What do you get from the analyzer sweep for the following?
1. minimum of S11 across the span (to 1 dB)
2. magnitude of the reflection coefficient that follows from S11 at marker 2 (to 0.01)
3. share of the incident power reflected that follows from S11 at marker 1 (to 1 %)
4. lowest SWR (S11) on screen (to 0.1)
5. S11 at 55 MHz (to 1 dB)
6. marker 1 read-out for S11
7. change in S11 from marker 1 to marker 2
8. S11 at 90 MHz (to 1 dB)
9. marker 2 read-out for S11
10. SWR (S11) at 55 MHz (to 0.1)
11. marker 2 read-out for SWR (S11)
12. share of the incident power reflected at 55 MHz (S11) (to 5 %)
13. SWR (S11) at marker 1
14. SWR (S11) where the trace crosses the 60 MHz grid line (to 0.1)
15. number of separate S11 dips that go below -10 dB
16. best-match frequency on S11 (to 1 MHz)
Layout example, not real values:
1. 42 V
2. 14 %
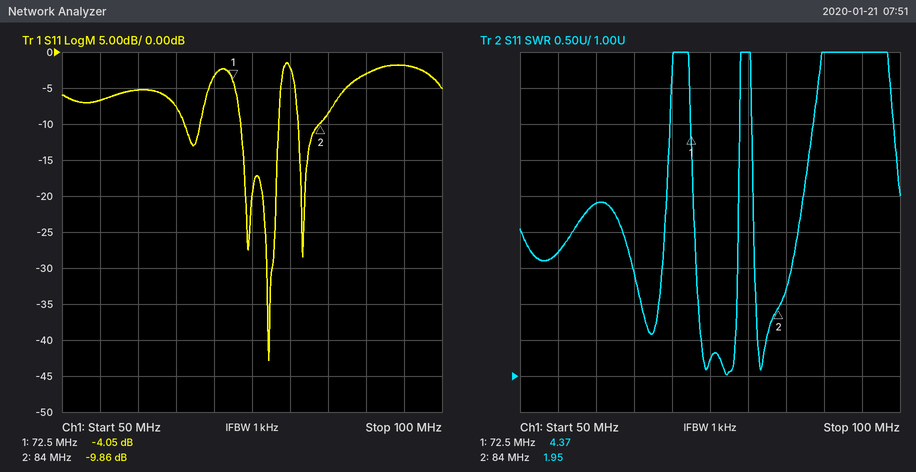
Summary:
1. -43 dB
2. 0.32
3. 39 %
4. 1.0
5. -7 dB
6. -4.05 dB
7. -5.81 dB
8. -3 dB
9. -9.86 dB
10. 2.7
11. 1.95
12. 20 %
13. 4.37
14. 3.4
15. 4
16. 77 MHz
